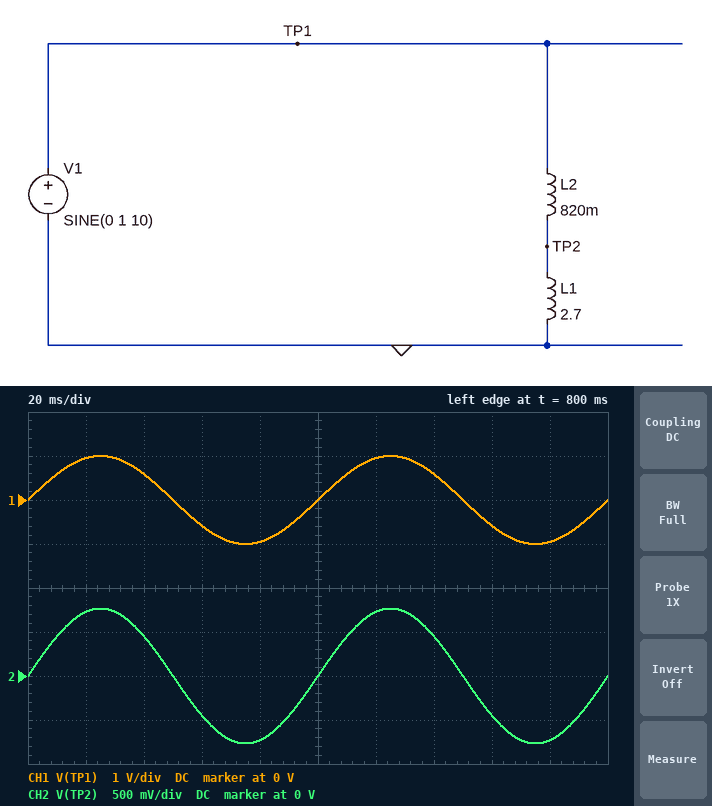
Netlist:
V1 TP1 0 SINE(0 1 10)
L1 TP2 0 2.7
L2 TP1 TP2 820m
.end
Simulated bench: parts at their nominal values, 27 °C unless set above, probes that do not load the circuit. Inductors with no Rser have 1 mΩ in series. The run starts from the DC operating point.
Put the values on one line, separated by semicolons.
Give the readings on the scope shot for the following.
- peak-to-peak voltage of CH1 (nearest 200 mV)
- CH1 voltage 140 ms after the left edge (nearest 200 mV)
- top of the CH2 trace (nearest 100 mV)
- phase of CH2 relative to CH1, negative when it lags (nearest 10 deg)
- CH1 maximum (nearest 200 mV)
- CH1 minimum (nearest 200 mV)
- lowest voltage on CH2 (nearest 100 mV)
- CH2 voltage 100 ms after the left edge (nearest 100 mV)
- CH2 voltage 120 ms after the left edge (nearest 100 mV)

2.0 V; 600 mV; 800 mV; 0 deg; 1.0 V; -1.0 V; -800 mV; 0 V; 700 mV
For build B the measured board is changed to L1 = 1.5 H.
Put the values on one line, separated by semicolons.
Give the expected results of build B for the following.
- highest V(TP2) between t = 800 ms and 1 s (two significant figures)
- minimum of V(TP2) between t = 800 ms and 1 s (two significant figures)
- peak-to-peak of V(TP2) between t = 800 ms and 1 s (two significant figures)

650 mV; -650 mV; 1.3 V
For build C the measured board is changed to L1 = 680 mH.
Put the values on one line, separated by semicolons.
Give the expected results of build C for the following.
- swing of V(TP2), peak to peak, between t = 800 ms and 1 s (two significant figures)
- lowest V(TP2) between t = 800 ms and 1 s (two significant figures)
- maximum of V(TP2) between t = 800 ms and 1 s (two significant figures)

910 mV; -450 mV; 450 mV
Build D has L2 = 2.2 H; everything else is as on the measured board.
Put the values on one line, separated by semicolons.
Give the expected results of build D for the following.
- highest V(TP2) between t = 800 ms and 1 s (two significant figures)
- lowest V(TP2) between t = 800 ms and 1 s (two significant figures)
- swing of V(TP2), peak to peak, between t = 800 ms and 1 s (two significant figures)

550 mV; -550 mV; 1.1 V
